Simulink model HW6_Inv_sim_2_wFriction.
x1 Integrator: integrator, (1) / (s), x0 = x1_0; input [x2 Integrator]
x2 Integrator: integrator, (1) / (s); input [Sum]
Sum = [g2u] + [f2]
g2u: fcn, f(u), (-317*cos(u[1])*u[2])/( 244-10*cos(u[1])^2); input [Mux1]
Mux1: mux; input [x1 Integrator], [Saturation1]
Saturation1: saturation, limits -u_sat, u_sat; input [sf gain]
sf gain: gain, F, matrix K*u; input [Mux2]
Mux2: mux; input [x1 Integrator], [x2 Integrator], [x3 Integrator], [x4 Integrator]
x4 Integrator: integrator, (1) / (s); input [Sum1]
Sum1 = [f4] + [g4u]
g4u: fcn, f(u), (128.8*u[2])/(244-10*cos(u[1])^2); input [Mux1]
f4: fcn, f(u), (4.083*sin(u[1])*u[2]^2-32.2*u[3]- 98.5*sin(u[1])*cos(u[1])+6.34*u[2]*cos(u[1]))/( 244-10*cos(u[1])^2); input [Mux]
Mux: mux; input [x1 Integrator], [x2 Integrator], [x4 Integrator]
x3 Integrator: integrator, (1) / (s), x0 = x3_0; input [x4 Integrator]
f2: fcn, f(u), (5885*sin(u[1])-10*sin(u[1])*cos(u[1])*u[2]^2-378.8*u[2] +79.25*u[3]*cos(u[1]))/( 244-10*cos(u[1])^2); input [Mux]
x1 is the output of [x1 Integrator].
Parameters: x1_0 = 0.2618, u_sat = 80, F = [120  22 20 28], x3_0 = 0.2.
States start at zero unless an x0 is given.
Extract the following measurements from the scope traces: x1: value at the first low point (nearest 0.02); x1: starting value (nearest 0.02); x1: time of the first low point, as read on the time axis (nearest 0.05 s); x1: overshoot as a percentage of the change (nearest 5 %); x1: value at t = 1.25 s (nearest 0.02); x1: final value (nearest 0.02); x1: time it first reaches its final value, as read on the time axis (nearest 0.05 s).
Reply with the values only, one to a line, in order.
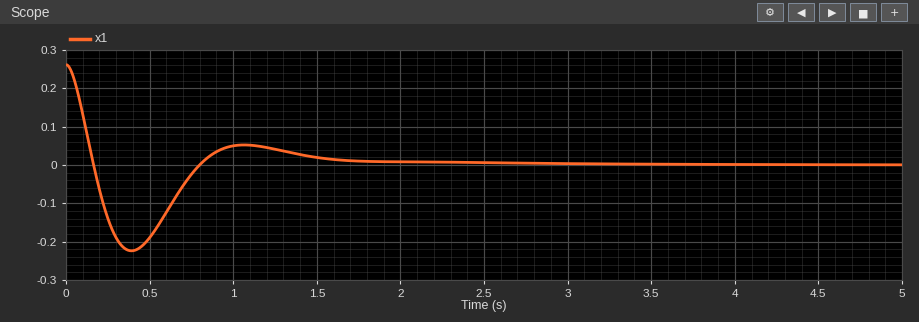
-0.22
0.26
0.40 s
85 %
0.04
0.00
0.15 s
